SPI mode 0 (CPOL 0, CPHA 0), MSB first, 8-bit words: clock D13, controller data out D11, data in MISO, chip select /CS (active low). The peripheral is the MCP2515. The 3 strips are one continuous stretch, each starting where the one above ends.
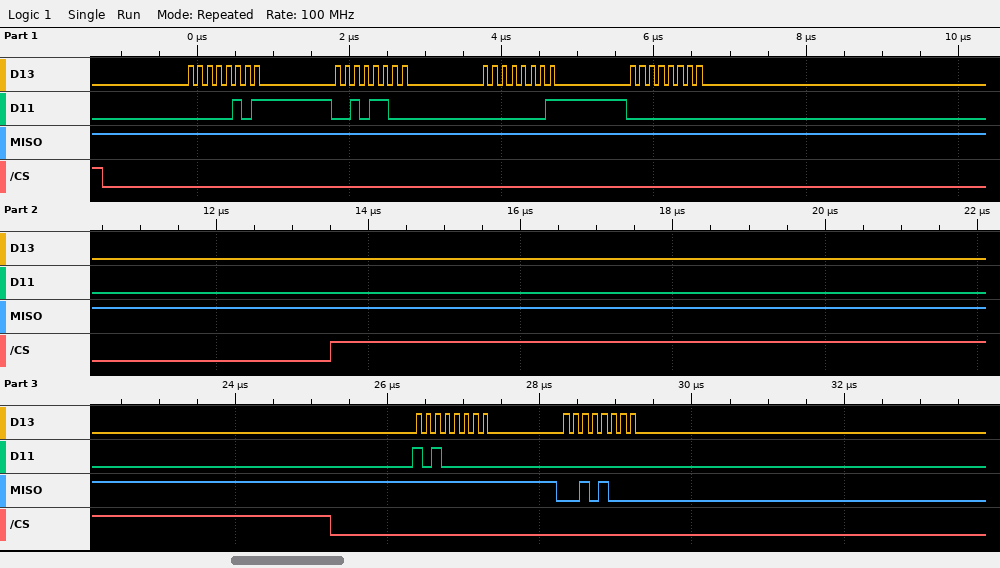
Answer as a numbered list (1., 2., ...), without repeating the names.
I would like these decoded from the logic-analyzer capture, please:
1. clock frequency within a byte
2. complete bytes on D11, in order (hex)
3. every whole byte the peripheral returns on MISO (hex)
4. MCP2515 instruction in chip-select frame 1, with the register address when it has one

1. 8 MHz
2. 05 2C 01 00 A0 00
3. FF FF FF FF FF 28
4. BIT MODIFY 0x2C
